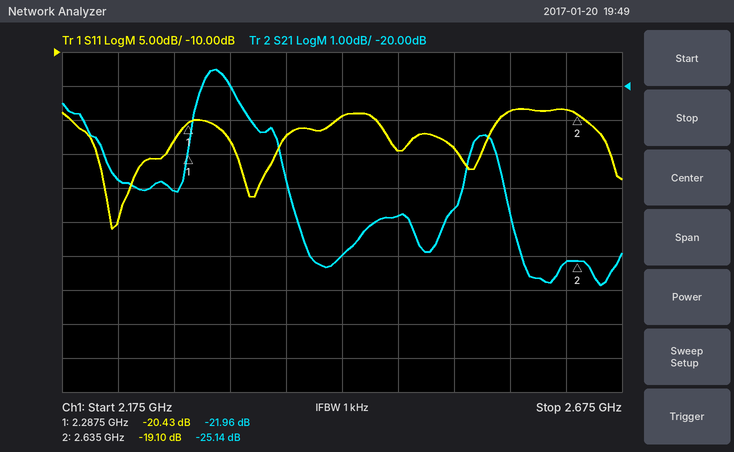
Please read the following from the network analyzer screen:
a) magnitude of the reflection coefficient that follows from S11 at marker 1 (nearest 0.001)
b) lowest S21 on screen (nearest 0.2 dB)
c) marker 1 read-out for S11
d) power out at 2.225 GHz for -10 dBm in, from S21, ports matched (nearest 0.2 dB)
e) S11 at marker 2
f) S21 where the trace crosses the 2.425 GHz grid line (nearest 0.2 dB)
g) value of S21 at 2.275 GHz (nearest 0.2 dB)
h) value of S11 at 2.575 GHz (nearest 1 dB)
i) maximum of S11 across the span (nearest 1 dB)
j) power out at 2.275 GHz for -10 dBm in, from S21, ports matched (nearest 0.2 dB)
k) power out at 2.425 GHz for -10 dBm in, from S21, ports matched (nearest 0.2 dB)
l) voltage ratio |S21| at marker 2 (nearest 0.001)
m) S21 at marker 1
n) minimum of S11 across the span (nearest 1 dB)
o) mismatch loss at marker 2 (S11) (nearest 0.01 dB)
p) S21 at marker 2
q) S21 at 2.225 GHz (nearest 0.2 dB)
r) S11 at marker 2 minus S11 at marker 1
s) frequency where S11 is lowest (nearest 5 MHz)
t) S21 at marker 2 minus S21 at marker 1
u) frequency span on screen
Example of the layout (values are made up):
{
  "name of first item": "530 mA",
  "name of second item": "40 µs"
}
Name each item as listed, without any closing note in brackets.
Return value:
{
  "magnitude of the reflection coefficient that follows from S11 at marker 1": "0.095",
  "lowest S21 on screen": "-25.8 dB",
  "marker 1 read-out for S11": "-20.43 dB",
  "power out at 2.225 GHz for -10 dBm in, from S21, ports matched": "-32.8 dBm",
  "S11 at marker 2": "-19.10 dB",
  "S21 where the trace crosses the 2.425 GHz grid line": "-25.0 dB",
  "value of S21 at 2.275 GHz": "-23.0 dB",
  "value of S11 at 2.575 GHz": "-19 dB",
  "maximum of S11 across the span": "-18 dB",
  "power out at 2.275 GHz for -10 dBm in, from S21, ports matched": "-33.0 dBm",
  "power out at 2.425 GHz for -10 dBm in, from S21, ports matched": "-35.0 dBm",
  "voltage ratio |S21| at marker 2": "0.055",
  "S21 at marker 1": "-21.96 dB",
  "minimum of S11 across the span": "-36 dB",
  "mismatch loss at marker 2 (S11)": "0.05 dB",
  "S21 at marker 2": "-25.14 dB",
  "S21 at 2.225 GHz": "-22.8 dB",
  "S11 at marker 2 minus S11 at marker 1": "1.33 dB",
  "frequency where S11 is lowest": "2.220 GHz",
  "S21 at marker 2 minus S21 at marker 1": "-3.18 dB",
  "frequency span on screen": "500 MHz"
}
